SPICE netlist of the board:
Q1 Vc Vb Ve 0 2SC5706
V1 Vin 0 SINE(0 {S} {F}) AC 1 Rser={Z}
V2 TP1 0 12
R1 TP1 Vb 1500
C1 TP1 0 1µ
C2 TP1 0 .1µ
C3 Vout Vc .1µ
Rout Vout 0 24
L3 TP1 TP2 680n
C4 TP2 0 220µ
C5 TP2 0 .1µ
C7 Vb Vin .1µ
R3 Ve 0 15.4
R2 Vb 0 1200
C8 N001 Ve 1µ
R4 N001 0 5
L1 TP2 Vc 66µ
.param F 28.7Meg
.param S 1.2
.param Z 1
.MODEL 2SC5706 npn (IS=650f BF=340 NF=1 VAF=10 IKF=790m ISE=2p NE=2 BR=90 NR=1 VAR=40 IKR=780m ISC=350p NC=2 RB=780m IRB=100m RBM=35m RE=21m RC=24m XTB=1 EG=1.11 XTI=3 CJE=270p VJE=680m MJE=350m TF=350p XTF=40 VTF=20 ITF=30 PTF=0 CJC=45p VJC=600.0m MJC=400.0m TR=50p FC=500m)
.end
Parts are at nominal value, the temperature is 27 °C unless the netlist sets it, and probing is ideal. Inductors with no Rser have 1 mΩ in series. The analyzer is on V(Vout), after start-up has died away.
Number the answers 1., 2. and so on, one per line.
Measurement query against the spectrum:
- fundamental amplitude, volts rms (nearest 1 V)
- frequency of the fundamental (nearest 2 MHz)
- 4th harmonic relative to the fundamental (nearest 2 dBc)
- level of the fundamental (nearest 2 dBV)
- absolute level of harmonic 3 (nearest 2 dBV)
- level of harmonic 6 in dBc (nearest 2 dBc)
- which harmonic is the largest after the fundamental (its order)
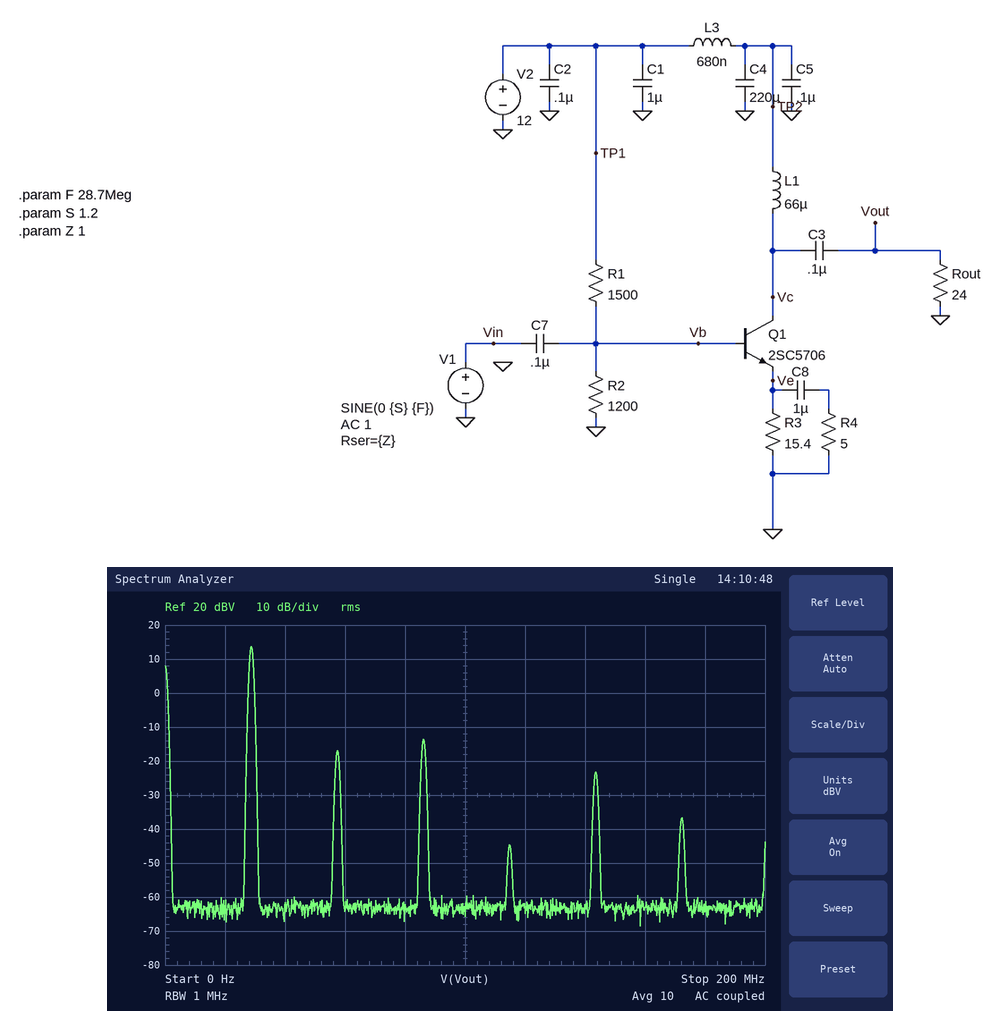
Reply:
1. 5 V
2. 28 MHz
3. -58 dBc
4. 14 dBV
5. -14 dBV
6. -50 dBc
7. 3
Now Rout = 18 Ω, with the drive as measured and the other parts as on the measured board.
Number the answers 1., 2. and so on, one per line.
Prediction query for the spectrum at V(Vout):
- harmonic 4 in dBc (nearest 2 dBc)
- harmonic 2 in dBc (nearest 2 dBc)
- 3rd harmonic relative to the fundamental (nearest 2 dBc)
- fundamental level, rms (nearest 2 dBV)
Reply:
1. -40 dBc
2. -34 dBc
3. -32 dBc
4. 12 dBV
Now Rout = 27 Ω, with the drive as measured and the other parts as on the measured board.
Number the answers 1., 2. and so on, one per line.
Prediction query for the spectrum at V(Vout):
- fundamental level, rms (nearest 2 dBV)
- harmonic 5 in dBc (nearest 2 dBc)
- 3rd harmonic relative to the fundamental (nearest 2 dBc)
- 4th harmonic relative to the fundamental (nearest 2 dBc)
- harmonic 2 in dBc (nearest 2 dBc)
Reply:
1. 14 dBV
2. -32 dBc
3. -24 dBc
4. -34 dBc
5. -26 dBc
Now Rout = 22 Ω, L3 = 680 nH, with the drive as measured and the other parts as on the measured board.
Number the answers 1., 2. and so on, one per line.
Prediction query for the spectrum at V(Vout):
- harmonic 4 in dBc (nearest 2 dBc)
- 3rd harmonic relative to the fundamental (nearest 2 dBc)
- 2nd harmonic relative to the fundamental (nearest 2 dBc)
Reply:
1. -46 dBc
2. -30 dBc
3. -32 dBc
